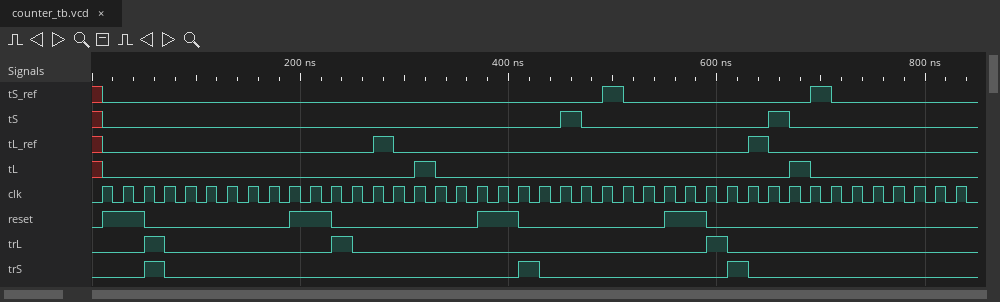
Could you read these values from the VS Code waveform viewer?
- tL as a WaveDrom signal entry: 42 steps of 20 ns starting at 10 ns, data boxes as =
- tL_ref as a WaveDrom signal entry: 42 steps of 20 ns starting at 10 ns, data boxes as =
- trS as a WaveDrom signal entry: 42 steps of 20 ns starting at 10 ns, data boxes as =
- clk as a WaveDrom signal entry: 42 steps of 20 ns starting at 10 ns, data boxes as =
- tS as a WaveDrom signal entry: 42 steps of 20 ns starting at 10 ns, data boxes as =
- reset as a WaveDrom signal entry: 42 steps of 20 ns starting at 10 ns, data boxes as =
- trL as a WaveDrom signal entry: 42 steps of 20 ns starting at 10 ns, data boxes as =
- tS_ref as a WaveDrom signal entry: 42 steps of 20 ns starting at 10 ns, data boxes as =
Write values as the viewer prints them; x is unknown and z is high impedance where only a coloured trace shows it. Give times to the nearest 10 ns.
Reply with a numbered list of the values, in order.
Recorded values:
1. {name: 'tL', wave: '0..............10................10.......'}
2. {name: 'tL_ref', wave: '0............10................10.........'}
3. {name: 'trS', wave: '0.10................10........10..........'}
4. {name: 'clk', wave: 'p.........................................'}
5. {name: 'tS', wave: '0.....................10........10........'}
6. {name: 'reset', wave: '1.0......1.0......1.0......1.0............'}
7. {name: 'trL', wave: '0.10.......10................10...........'}
8. {name: 'tS_ref', wave: '0.......................10........10......'}
